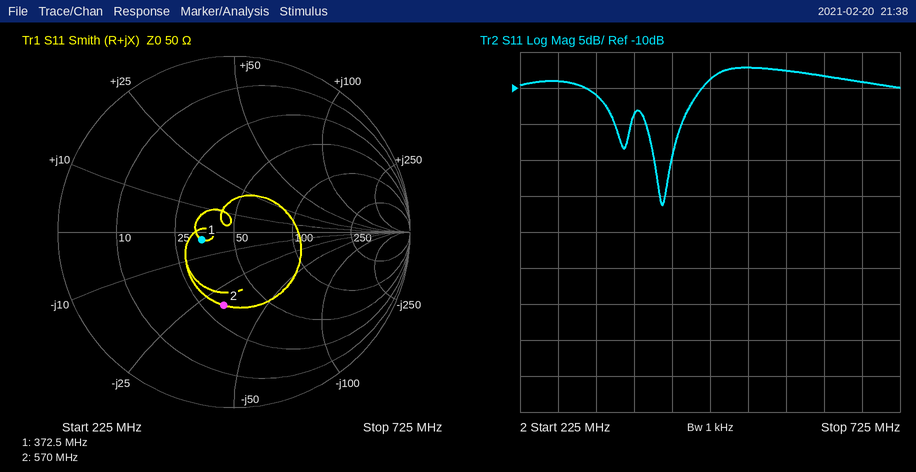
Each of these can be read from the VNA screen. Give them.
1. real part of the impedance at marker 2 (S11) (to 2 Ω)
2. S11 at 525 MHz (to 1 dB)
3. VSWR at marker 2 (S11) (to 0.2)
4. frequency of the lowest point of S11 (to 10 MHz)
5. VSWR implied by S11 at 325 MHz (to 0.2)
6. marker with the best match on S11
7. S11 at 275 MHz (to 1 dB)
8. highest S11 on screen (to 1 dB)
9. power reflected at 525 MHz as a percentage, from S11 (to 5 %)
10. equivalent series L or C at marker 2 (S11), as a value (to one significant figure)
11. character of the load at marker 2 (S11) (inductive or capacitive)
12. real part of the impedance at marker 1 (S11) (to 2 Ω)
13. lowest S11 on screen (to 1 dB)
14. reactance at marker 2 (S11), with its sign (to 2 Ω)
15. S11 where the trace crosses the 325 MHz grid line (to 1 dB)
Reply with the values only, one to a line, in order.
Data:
32 Ω
-7 dB
2.4
410 MHz
1.8
marker 1
-9 dB
-7 dB
20 %
9 pF
capacitive
34 Ω
-26 dB
-32 Ω
-11 dB
